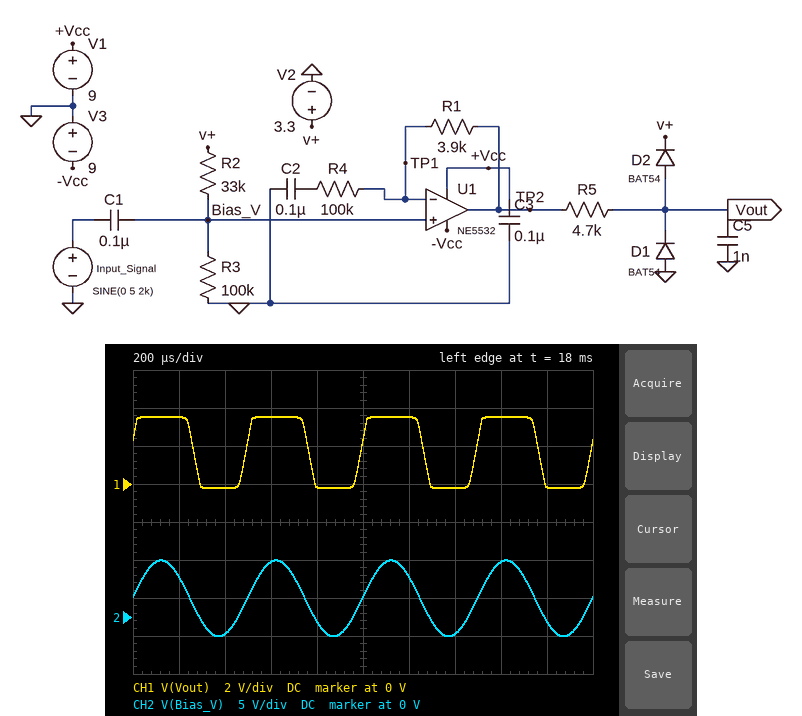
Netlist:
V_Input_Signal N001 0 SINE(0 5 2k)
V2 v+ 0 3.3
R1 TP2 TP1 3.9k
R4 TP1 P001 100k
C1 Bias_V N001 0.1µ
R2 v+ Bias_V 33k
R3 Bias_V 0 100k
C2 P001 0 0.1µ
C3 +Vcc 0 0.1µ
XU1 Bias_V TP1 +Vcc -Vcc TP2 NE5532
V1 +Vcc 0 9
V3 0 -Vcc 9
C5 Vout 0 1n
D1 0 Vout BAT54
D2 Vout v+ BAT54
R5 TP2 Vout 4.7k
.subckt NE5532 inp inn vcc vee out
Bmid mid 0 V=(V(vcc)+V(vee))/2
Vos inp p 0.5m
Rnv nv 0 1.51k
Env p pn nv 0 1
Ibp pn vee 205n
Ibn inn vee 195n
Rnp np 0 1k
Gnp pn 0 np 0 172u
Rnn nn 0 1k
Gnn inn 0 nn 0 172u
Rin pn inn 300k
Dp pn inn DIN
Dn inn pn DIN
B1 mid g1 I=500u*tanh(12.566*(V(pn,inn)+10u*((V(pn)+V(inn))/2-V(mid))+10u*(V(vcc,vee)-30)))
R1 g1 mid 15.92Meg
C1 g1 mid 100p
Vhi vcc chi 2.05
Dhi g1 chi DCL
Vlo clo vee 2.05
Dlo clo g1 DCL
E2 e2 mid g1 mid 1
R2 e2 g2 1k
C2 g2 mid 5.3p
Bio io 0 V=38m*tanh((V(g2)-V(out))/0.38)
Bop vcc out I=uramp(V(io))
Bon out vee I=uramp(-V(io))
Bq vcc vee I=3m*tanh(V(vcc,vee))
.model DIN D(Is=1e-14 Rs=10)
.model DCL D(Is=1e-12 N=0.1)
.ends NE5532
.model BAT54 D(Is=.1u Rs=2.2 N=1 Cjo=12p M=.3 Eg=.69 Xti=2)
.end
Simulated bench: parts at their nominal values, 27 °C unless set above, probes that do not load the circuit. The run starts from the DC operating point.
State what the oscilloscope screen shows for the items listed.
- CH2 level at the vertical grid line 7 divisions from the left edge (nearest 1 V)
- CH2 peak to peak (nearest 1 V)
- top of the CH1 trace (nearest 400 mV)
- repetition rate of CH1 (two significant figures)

-2 V
10 V
3.6 V
2.0 kHz
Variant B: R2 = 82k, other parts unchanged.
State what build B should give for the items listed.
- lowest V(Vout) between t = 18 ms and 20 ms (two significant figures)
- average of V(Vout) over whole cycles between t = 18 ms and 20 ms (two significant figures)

-230 mV
1.7 V
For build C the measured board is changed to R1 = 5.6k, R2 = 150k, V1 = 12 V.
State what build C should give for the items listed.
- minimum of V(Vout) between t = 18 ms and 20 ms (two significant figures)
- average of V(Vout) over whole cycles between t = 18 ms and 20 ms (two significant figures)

-230 mV
1.6 V
